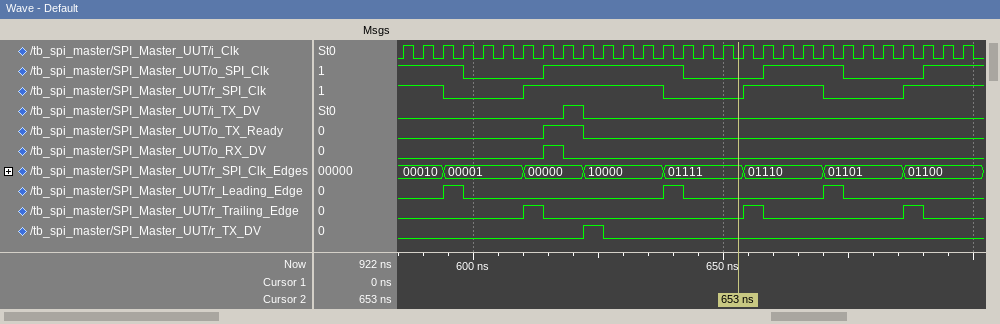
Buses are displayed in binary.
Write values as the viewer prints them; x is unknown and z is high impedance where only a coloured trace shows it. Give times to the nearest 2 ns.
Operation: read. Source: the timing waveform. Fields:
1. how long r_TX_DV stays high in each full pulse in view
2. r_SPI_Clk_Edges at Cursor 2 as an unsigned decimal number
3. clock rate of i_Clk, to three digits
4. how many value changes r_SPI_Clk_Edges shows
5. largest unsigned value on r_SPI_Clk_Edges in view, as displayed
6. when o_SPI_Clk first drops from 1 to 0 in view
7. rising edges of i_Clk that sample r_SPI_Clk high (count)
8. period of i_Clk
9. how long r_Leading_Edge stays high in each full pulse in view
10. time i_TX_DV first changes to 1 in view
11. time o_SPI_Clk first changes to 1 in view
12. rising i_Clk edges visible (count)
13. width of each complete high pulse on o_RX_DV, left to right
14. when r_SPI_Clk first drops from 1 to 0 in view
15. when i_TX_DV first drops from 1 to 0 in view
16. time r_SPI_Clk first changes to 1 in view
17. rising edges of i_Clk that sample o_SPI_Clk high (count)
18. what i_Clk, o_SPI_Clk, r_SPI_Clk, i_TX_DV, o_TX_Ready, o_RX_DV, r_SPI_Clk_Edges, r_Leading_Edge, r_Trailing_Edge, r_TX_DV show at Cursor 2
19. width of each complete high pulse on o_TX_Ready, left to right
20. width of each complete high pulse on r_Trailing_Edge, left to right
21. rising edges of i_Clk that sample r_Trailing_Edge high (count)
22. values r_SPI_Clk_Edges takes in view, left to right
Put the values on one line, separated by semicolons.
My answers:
4 ns; 15; 250 MHz; 7; 10000; 598 ns; 17; 4 ns; 4 ns, 4 ns, 4 ns; 618 ns; 614 ns; 29; 4 ns; 594 ns; 622 ns; 610 ns; 17; i_Clk=0, o_SPI_Clk=0, r_SPI_Clk=0, i_TX_DV=0, o_TX_Ready=0, o_RX_DV=0, r_SPI_Clk_Edges=01111, r_Leading_Edge=0, r_Trailing_Edge=0, r_TX_DV=0; 8 ns; 4 ns, 4 ns, 4 ns; 3; 00010, 00001, 00000, 10000, 01111, 01110, 01101, 01100
